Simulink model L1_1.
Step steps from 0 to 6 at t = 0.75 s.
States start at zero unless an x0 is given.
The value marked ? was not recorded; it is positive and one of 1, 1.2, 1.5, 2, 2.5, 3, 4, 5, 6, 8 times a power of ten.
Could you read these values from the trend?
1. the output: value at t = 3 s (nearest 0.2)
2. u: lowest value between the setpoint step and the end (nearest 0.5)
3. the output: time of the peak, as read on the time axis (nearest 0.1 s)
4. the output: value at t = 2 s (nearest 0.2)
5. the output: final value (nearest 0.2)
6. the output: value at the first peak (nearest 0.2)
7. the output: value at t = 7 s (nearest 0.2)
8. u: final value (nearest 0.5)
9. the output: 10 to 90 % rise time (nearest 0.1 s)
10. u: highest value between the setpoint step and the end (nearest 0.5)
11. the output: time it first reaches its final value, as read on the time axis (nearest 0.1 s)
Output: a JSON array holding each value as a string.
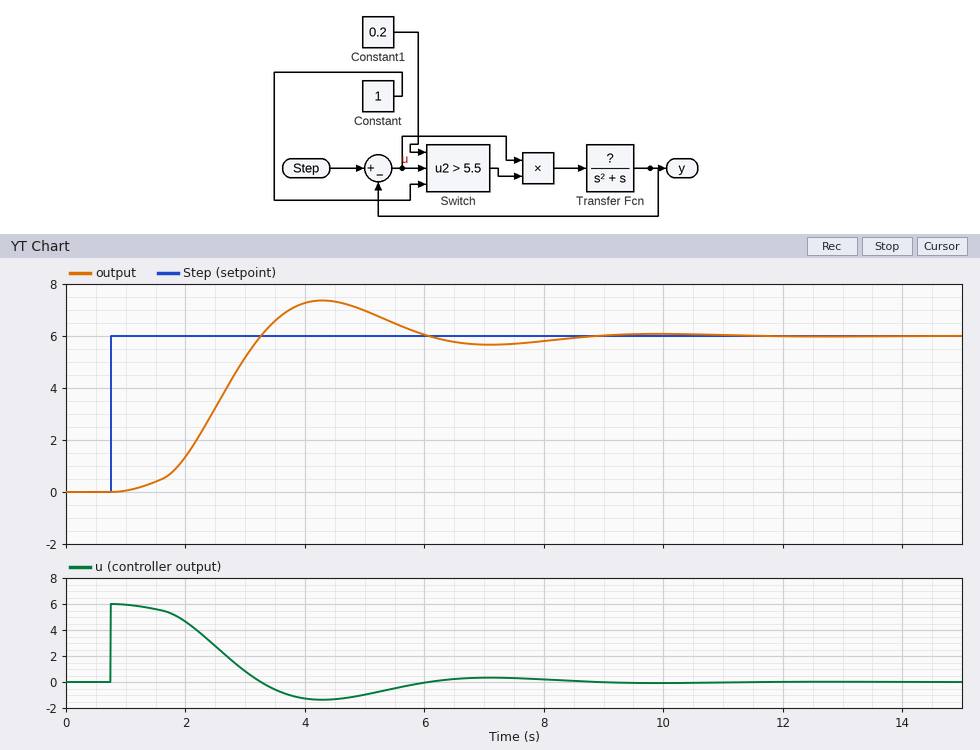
["5.2", "-1.5", "4.3 s", "1.4", "6.0", "7.4", "5.6", "0.0", "1.4 s", "6.0", "3.3 s"]
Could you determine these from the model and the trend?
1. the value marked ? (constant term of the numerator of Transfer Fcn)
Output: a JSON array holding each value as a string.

["1.5"]
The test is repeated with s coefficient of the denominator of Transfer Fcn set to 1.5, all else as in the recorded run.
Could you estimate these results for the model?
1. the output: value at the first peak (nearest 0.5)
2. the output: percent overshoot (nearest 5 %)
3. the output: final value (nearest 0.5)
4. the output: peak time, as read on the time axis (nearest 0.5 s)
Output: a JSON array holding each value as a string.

["6.5", "10 %", "6.0", "5.0 s"]
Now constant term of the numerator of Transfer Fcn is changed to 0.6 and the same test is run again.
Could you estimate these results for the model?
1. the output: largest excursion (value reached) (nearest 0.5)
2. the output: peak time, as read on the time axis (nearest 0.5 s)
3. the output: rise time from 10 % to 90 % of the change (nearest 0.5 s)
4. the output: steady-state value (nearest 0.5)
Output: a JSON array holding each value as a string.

["6.5", "7.5 s", "3.0 s", "6.0"]
